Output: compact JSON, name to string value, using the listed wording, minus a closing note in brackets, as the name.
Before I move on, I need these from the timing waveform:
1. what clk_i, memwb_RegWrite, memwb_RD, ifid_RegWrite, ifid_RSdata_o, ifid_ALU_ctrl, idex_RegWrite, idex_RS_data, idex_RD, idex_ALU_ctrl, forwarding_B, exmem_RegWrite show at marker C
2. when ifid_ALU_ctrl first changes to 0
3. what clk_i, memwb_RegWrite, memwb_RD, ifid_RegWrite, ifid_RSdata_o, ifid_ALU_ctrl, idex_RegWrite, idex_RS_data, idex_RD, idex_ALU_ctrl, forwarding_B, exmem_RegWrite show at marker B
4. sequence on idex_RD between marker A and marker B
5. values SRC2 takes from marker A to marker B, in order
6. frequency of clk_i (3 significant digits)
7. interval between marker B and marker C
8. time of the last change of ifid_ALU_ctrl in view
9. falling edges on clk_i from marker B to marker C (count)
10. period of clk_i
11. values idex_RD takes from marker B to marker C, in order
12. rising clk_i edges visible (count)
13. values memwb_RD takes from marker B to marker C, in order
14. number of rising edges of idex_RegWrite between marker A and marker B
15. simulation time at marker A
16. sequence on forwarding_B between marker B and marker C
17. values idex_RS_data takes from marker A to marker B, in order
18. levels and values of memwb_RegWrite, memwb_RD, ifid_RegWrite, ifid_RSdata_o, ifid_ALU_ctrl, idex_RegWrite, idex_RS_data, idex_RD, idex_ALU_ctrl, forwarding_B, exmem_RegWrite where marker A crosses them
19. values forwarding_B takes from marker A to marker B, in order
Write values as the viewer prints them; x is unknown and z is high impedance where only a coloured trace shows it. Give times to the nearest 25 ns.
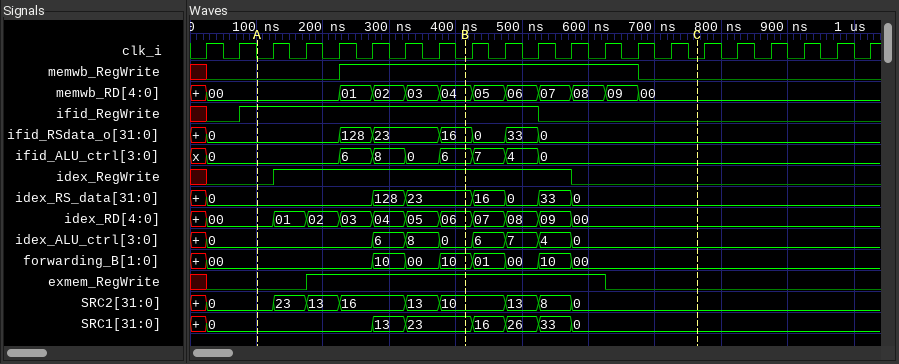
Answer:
{"what clk_i, memwb_RegWrite, memwb_RD, ifid_RegWrite, ifid_RSdata_o, ifid_ALU_ctrl, idex_RegWrite, idex_RS_data, idex_RD, idex_ALU_ctrl, forwarding_B, exmem_RegWrite show at marker C": "clk_i=0, memwb_RegWrite=0, memwb_RD=00, ifid_RegWrite=0, ifid_RSdata_o=0, ifid_ALU_ctrl=0, idex_RegWrite=0, idex_RS_data=0, idex_RD=00, idex_ALU_ctrl=0, forwarding_B=00, exmem_RegWrite=0", "when ifid_ALU_ctrl first changes to 0": "25 ns", "what clk_i, memwb_RegWrite, memwb_RD, ifid_RegWrite, ifid_RSdata_o, ifid_ALU_ctrl, idex_RegWrite, idex_RS_data, idex_RD, idex_ALU_ctrl, forwarding_B, exmem_RegWrite show at marker B": "clk_i=0, memwb_RegWrite=1, memwb_RD=04, ifid_RegWrite=1, ifid_RSdata_o=16, ifid_ALU_ctrl=6, idex_RegWrite=1, idex_RS_data=23, idex_RD=06, idex_ALU_ctrl=0, forwarding_B=10, exmem_RegWrite=1", "sequence on idex_RD between marker A and marker B": "00, 01, 02, 03, 04, 05, 06", "values SRC2 takes from marker A to marker B, in order": "0, 23, 13, 16, 13, 10", "frequency of clk_i": "20.0 MHz", "interval between marker B and marker C": "350 ns", "time of the last change of ifid_ALU_ctrl in view": "525 ns", "falling edges on clk_i from marker B to marker C": "7", "period of clk_i": "50 ns", "values idex_RD takes from marker B to marker C, in order": "06, 07, 08, 09, 00", "rising clk_i edges visible": "21", "values memwb_RD takes from marker B to marker C, in order": "04, 05, 06, 07, 08, 09, 00", "number of rising edges of idex_RegWrite between marker A and marker B": "1", "simulation time at marker A": "100 ns", "sequence on forwarding_B between marker B and marker C": "10, 01, 00, 10, 00", "values idex_RS_data takes from marker A to marker B, in order": "0, 128, 23", "levels and values of memwb_RegWrite, memwb_RD, ifid_RegWrite, ifid_RSdata_o, ifid_ALU_ctrl, idex_RegWrite, idex_RS_data, idex_RD, idex_ALU_ctrl, forwarding_B, exmem_RegWrite where marker A crosses them": "memwb_RegWrite=0, memwb_RD=00, ifid_RegWrite=1, ifid_RSdata_o=0, ifid_ALU_ctrl=0, idex_RegWrite=0, idex_RS_data=0, idex_RD=00, idex_ALU_ctrl=0, forwarding_B=00, exmem_RegWrite=0", "values forwarding_B takes from marker A to marker B, in order": "00, 10, 00, 10"}
